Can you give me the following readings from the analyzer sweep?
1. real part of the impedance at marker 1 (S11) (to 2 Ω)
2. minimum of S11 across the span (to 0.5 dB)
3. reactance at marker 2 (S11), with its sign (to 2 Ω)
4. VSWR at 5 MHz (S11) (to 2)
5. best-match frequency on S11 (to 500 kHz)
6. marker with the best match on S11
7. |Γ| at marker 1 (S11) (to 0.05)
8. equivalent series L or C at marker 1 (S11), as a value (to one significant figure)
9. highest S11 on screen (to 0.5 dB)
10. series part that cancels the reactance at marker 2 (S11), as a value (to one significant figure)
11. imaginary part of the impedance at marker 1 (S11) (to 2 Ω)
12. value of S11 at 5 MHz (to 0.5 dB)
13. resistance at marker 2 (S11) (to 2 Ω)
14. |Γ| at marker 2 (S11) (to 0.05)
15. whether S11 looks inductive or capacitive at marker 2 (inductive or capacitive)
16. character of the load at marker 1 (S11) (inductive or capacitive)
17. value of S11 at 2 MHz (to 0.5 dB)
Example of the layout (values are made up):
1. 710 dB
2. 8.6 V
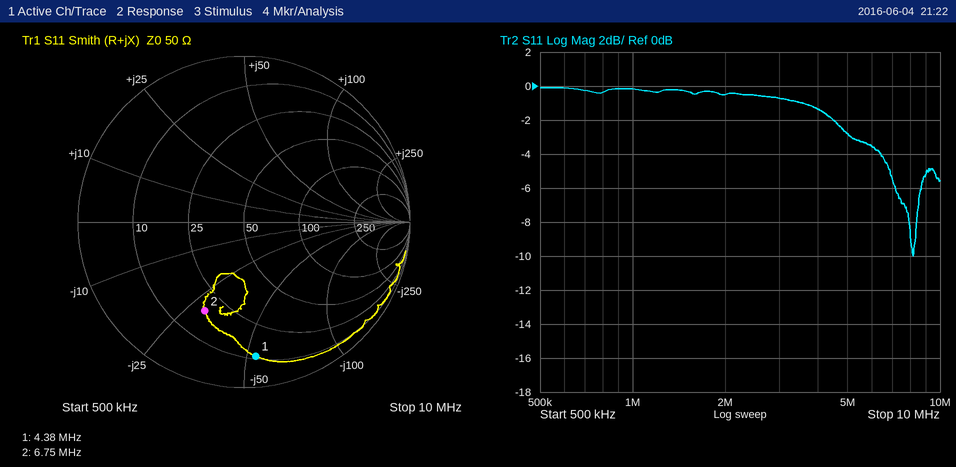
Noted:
1. 12 Ω
2. -10.0 dB
3. -30 Ω
4. 6
5. 8.0 MHz
6. marker 2
7. 0.80
8. 700 pF
9. 0.0 dB
10. 700 nH
11. -54 Ω
12. -3.0 dB
13. 18 Ω
14. 0.60
15. capacitive
16. capacitive
17. -0.5 dB
